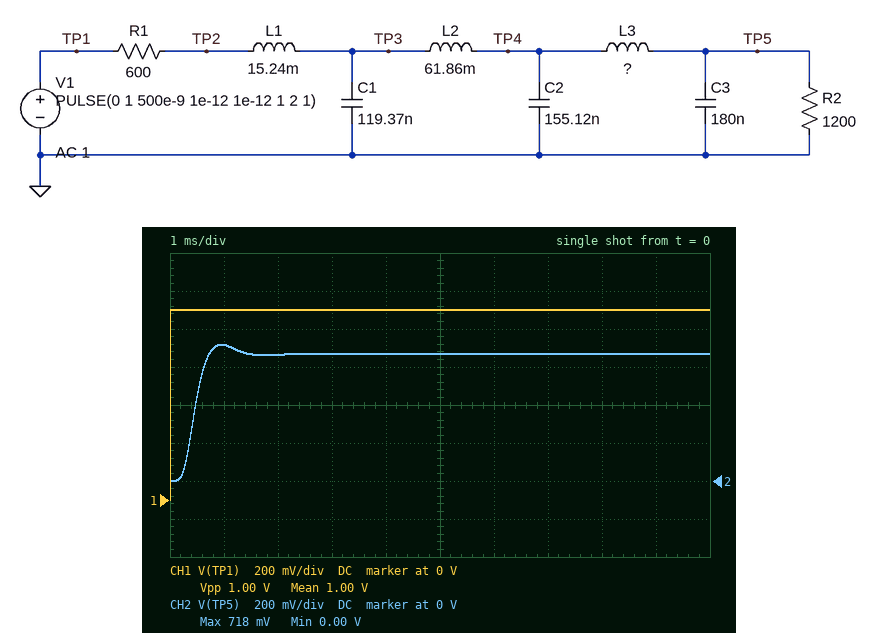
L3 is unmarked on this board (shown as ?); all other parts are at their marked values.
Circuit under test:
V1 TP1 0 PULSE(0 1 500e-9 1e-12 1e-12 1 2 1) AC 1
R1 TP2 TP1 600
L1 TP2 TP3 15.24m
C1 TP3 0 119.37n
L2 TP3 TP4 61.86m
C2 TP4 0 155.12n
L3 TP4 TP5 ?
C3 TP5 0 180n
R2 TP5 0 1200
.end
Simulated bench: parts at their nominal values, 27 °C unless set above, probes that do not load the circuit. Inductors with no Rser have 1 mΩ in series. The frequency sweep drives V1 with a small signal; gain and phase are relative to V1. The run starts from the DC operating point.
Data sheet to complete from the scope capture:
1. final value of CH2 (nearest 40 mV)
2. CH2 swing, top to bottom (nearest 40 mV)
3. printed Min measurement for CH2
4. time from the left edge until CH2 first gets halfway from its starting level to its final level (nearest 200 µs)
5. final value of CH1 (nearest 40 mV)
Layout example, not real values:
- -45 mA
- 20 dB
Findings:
- 680 mV
- 720 mV
- 0.00 V
- 400 µs
- 1.00 V
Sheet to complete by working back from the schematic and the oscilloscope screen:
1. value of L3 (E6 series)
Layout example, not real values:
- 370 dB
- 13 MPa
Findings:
- 330 mH
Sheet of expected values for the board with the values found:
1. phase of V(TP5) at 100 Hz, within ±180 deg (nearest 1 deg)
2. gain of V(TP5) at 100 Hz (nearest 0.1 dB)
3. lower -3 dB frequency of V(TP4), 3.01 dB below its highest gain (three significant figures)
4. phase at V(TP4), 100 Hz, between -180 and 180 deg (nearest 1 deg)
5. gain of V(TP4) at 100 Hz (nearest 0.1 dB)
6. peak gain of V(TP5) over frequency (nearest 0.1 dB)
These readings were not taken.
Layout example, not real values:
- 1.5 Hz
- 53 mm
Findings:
- -15 deg
- -3.5 dB
- 763 Hz
- -5 deg
- -3.6 dB
- -3.3 dB
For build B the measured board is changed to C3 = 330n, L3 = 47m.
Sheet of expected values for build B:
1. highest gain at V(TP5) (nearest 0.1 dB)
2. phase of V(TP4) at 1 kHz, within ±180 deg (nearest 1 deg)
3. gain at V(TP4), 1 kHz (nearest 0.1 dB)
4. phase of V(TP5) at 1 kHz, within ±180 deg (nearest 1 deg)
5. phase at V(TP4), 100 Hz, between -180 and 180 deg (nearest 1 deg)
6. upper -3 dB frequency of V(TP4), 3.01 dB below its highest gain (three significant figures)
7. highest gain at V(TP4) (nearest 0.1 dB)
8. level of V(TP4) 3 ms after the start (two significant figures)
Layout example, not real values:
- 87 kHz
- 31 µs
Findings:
- -3.5 dB
- -77 deg
- -12.0 dB
- -110 deg
- -10 deg
- 3.06 kHz
- 4.1 dB
- 670 mV
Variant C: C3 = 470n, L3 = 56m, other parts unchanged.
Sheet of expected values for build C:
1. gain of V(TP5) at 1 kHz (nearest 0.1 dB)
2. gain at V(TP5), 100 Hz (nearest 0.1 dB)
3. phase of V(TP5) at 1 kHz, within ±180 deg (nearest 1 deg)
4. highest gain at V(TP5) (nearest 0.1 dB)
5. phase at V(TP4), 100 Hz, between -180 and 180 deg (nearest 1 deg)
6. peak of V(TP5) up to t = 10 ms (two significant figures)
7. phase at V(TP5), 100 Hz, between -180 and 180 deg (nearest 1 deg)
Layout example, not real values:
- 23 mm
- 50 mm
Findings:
- -6.7 dB
- -3.6 dB
- -126 deg
- -3.5 dB
- -12 deg
- 670 mV
- -13 deg
